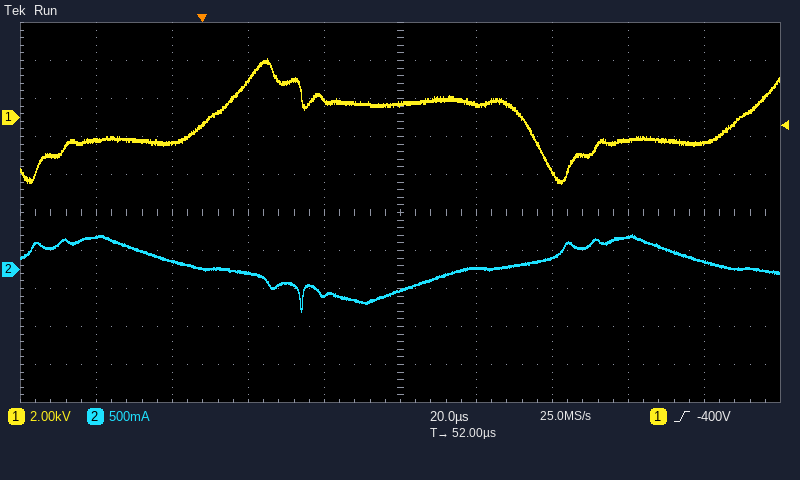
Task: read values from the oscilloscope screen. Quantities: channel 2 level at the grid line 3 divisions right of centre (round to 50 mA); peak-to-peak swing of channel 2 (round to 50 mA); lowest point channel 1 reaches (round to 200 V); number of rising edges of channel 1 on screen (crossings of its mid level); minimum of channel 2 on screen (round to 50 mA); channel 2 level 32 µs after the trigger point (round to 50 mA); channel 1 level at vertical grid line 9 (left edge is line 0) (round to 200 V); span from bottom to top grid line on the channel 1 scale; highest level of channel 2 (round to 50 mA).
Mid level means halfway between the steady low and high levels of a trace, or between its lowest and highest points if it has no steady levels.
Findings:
450 mA
1.00 A
-3.4 kV
2
-550 mA
-350 mA
-1.4 kV
20 kV
450 mA
